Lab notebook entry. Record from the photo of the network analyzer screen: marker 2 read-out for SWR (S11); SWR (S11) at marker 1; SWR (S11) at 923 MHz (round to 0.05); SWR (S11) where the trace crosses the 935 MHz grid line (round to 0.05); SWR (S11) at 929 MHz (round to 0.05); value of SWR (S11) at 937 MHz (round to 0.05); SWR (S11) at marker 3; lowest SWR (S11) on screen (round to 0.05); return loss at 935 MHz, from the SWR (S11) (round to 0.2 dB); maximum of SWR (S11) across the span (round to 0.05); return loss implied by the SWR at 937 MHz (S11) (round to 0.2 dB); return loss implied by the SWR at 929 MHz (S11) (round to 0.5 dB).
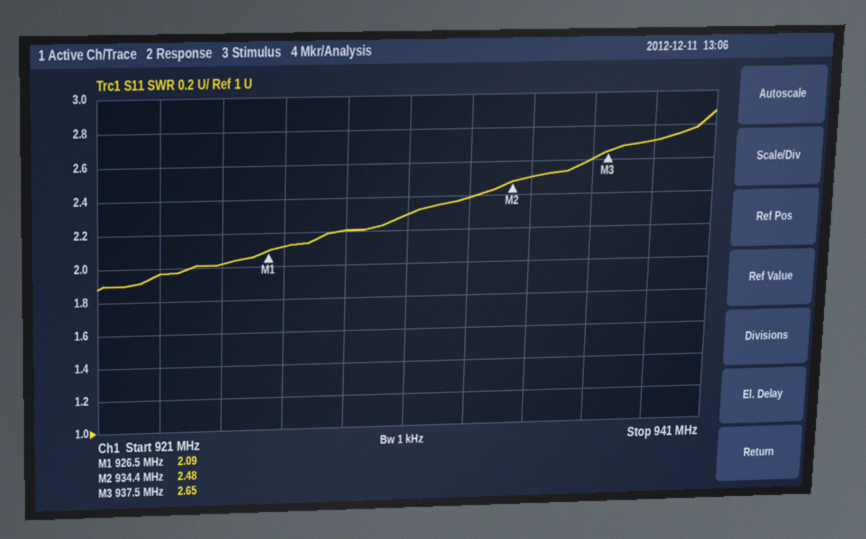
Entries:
2.48
2.09
1.95
2.50
2.20
2.60
2.65
1.90
7.4 dB
2.90
7.0 dB
8.5 dB
